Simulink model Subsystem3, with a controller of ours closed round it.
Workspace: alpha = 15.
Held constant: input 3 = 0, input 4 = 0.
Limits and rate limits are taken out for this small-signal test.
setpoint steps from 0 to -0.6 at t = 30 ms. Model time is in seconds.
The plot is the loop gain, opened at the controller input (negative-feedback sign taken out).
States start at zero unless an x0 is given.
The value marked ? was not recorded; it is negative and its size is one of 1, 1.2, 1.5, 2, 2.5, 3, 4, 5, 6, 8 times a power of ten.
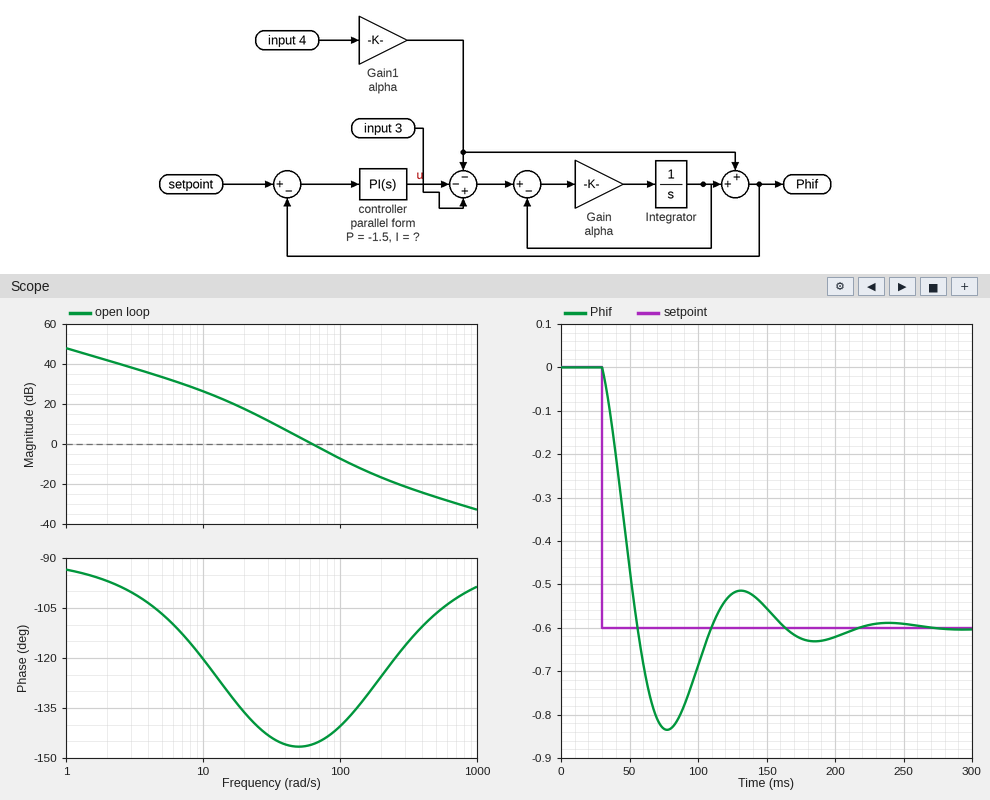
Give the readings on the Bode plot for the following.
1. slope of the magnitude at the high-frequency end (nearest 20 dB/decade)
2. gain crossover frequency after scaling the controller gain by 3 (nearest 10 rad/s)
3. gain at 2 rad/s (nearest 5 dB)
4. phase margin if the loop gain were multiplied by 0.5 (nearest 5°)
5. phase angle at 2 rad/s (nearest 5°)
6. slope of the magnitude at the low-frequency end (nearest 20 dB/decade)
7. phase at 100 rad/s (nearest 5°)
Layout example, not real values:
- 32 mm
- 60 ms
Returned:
- -20 dB/decade
- 120 rad/s
- 40 dB
- 35°
- -95°
- -20 dB/decade
- -140°
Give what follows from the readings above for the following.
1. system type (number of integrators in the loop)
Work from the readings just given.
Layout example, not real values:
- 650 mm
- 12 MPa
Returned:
- 1
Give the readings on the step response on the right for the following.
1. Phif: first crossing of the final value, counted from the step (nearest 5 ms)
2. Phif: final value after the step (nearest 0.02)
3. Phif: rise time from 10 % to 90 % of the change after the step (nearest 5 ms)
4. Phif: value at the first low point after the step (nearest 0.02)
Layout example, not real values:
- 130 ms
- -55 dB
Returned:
- 25 ms
- -0.60
- 20 ms
- -0.84
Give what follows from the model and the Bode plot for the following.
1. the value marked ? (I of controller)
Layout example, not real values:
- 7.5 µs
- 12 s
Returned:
- -250
